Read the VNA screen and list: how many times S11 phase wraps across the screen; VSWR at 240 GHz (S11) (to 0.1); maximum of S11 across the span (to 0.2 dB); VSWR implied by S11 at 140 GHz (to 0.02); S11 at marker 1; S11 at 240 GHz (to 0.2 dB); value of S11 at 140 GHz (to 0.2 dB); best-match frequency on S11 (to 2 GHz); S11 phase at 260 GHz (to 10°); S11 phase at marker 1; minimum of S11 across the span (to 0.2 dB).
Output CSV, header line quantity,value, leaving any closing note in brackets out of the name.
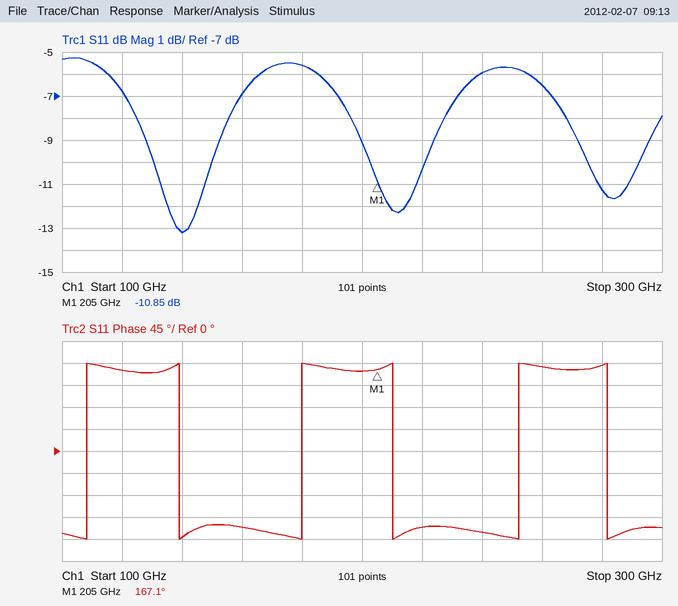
quantity,value
how many times S11 phase wraps across the screen,6
VSWR at 240 GHz (S11),3.0
maximum of S11 across the span,-5.2 dB
VSWR implied by S11 at 140 GHz,1.56
S11 at marker 1,-10.85 dB
S11 at 240 GHz,-6.0 dB
value of S11 at 140 GHz,-13.2 dB
best-match frequency on S11,140 GHz
S11 phase at 260 GHz,170°
S11 phase at marker 1,167.1°
minimum of S11 across the span,-13.2 dB
